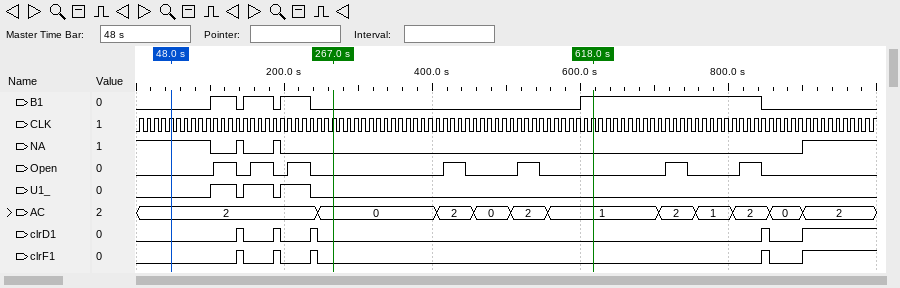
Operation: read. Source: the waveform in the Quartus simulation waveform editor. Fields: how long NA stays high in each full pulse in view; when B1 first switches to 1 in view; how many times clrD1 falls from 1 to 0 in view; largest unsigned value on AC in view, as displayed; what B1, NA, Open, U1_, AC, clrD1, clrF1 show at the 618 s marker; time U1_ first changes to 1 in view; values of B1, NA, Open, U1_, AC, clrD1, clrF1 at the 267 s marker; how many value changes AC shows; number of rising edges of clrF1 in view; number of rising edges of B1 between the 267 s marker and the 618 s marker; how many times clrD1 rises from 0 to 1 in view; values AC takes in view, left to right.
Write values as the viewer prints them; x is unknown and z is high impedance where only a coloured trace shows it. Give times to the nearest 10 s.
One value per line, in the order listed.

10 s, 10 s
100 s
4
2
B1=1, NA=0, Open=0, U1_=0, AC=1, clrD1=0, clrF1=0
100 s
B1=0, NA=0, Open=0, U1_=0, AC=0, clrD1=0, clrF1=0
10
5
1
5
2, 0, 2, 0, 2, 1, 2, 1, 2, 0, 2
